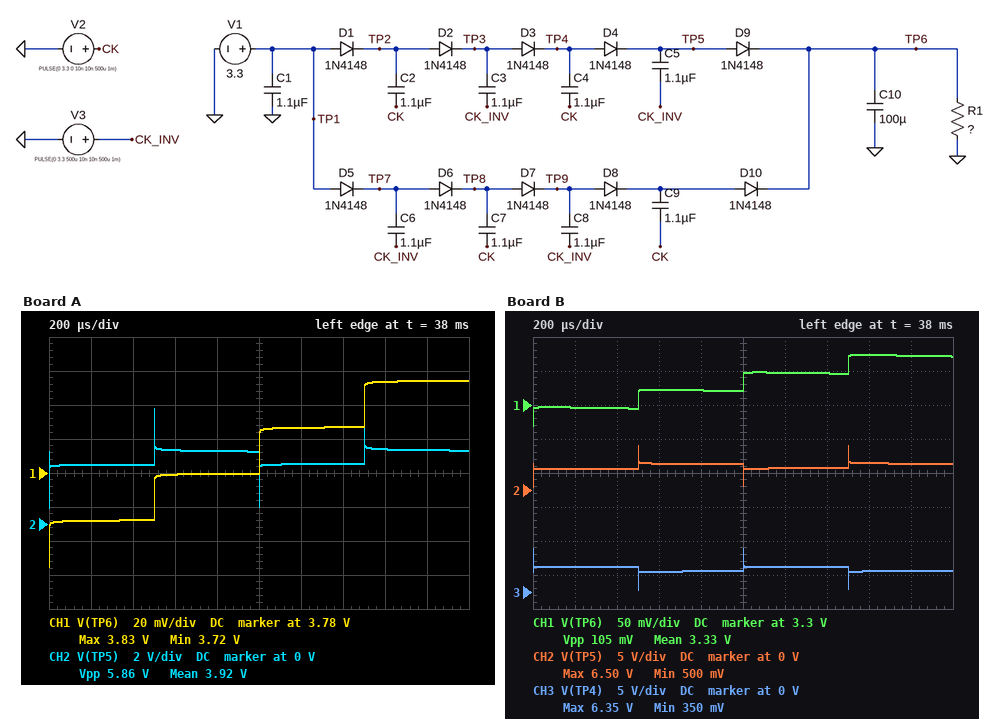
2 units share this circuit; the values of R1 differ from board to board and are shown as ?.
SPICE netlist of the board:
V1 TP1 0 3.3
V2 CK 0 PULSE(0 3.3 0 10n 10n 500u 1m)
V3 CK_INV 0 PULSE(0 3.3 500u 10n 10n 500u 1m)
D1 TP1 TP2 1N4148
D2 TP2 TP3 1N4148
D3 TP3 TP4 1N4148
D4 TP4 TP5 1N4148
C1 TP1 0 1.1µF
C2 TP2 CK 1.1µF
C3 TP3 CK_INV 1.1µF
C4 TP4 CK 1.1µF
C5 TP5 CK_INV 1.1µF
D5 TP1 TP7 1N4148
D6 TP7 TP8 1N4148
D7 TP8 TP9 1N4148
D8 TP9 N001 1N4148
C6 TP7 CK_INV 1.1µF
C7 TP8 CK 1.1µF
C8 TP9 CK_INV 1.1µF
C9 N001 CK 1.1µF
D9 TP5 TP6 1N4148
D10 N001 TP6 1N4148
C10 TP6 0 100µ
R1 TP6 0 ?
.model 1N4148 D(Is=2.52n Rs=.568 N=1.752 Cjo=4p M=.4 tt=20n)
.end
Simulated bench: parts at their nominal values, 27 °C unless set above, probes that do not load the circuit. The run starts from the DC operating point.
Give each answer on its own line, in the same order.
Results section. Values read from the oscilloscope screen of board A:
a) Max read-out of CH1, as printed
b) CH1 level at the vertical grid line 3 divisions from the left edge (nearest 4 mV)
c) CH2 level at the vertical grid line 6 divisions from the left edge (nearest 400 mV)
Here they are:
3.83 V
3.780 V
3.6 V
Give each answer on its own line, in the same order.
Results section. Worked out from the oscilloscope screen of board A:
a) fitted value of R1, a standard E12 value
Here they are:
39 kΩ
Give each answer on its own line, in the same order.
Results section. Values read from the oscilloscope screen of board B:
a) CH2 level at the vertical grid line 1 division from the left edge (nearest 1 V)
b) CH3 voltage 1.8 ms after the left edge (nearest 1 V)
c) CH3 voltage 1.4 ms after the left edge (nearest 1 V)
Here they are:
3 V
3 V
4 V
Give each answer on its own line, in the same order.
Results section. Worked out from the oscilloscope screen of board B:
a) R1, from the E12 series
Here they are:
4.7 kΩ
